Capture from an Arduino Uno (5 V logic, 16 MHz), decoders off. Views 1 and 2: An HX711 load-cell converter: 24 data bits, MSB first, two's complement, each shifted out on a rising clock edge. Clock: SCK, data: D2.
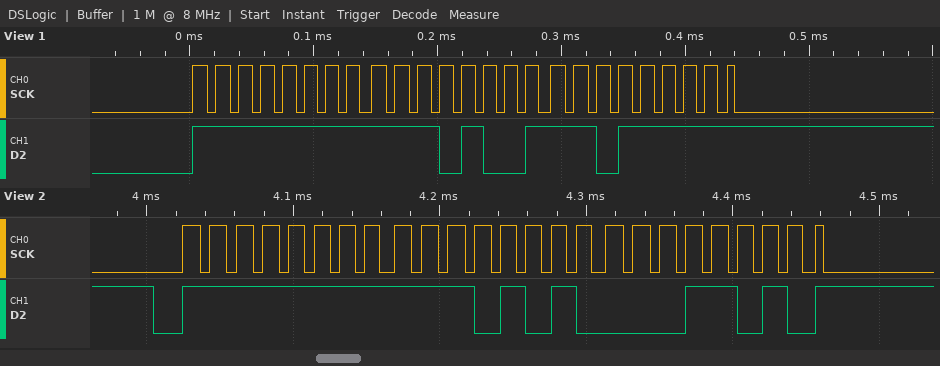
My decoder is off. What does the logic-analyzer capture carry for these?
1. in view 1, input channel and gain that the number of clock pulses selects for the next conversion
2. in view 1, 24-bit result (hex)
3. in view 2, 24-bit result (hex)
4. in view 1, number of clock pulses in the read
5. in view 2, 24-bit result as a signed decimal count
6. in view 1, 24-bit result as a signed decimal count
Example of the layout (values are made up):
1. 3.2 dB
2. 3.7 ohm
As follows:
1. channel A, gain 128
2. 0xFFE9DF
3. 0xFFEA1A
4. 25
5. -5606
6. -5665
